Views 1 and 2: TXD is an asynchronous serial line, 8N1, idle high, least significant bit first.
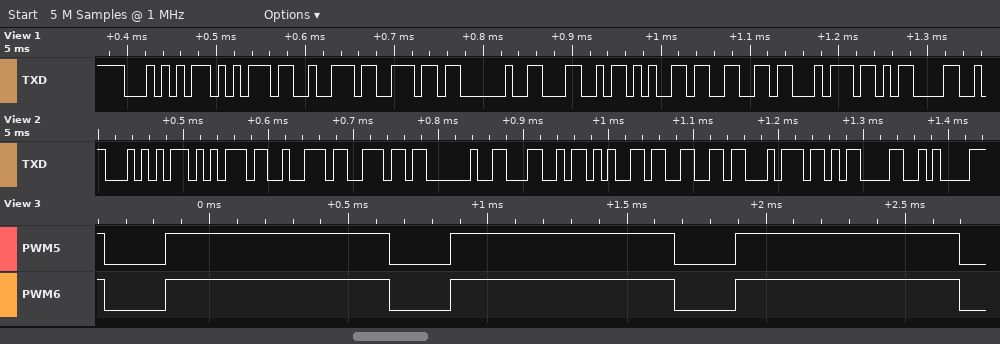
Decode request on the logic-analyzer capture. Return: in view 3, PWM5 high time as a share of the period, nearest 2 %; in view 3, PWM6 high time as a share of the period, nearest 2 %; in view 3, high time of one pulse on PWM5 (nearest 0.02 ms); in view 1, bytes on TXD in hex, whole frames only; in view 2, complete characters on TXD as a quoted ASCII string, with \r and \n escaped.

78 %
78 %
0.80 ms
54 75 72 6E 20 4C 65 66 74 0D
"Turn Left\r\n"
